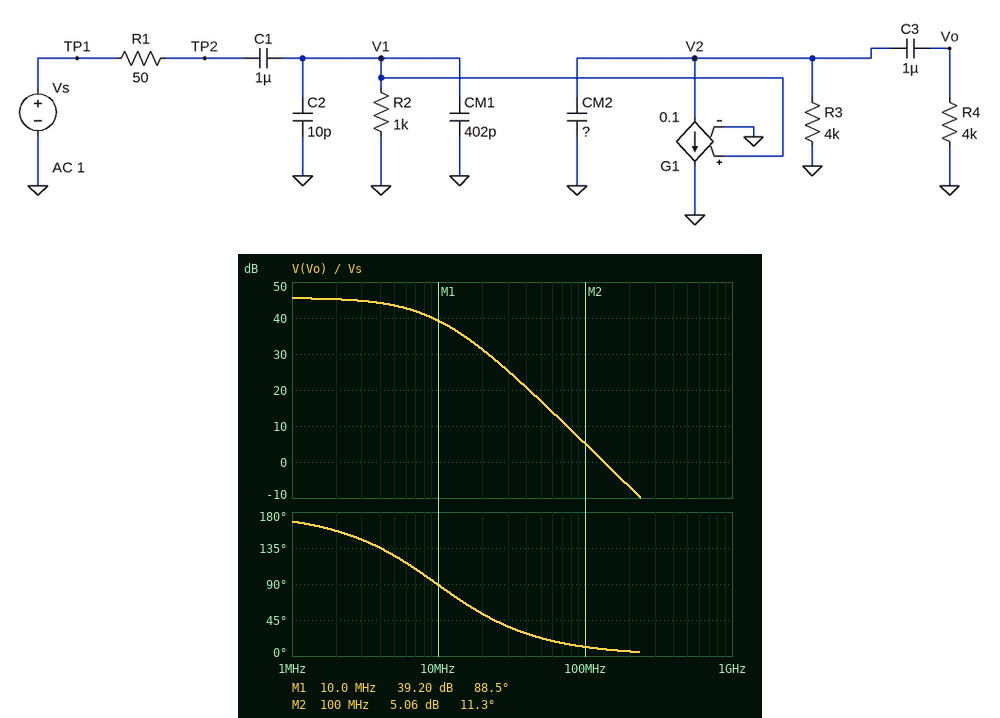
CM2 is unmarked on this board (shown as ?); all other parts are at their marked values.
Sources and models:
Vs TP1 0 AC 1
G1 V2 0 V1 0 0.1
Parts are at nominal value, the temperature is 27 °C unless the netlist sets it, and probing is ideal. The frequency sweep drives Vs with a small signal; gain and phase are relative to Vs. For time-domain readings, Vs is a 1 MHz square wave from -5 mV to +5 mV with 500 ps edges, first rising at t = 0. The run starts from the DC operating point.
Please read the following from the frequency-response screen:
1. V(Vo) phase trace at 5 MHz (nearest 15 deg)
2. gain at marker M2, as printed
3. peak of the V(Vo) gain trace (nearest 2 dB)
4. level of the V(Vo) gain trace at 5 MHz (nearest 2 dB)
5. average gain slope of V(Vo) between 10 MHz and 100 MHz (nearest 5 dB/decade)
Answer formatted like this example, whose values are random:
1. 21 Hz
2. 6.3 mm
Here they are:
1. 120 deg
2. 5.06 dB
3. 46 dB
4. 44 dB
5. -35 dB/decade
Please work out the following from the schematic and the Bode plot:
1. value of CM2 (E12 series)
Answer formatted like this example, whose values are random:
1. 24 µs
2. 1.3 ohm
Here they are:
1. 6.8 pF
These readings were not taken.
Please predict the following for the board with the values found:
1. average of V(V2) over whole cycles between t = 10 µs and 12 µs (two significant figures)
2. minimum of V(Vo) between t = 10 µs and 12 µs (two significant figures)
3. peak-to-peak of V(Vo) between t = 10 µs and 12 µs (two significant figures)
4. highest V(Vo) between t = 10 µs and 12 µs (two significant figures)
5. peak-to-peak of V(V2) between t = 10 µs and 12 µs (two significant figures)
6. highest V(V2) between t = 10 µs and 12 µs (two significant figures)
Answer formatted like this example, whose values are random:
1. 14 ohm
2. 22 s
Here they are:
1. -940 mV
2. -1.9 V
3. 1.9 V
4. 12 mV
5. 1.9 V
6. 9.4 mV
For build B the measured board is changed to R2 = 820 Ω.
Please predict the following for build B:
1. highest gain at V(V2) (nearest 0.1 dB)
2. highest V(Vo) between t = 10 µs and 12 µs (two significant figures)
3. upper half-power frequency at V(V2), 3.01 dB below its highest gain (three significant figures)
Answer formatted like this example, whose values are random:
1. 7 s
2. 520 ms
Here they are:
1. 45.5 dB
2. 14 mV
3. 6.17 MHz
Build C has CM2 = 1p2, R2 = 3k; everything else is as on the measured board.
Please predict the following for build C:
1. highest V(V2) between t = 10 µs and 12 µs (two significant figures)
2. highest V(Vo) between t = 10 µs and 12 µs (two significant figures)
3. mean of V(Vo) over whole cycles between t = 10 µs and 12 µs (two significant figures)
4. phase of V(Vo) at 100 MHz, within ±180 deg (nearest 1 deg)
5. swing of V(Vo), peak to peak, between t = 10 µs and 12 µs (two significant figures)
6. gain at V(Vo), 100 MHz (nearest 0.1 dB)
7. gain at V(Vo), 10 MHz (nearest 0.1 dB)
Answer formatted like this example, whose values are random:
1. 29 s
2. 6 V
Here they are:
1. 2.4 mV
2. 5.3 mV
3. -980 mV
4. 38 deg
5. 2.0 V
6. 18.6 dB
7. 41.6 dB
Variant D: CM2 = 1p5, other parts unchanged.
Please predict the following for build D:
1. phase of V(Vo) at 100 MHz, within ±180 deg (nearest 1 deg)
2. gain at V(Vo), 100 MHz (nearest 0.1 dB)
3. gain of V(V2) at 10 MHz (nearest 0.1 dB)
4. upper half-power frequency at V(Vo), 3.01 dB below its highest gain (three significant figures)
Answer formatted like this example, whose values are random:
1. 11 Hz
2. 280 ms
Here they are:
1. 33 deg
2. 17.2 dB
3. 41.4 dB
4. 7.94 MHz
